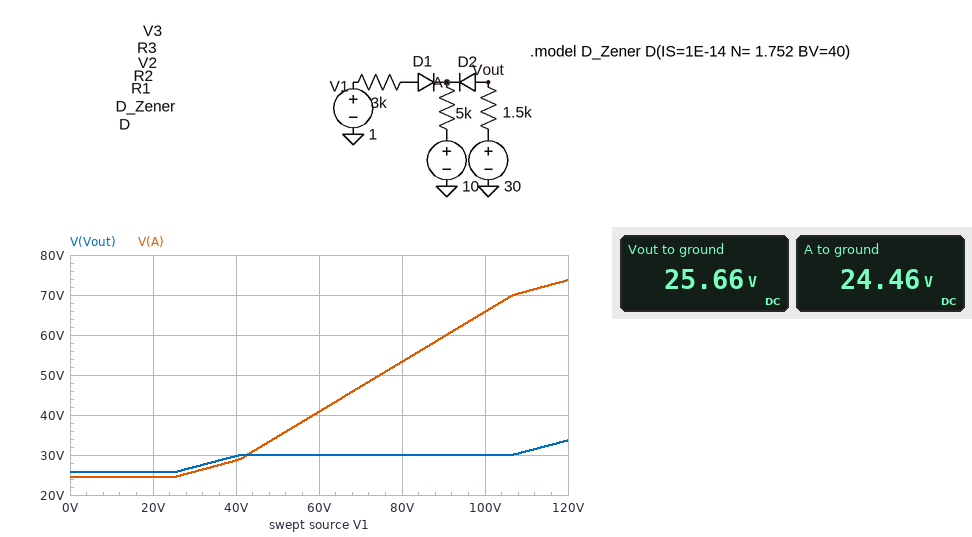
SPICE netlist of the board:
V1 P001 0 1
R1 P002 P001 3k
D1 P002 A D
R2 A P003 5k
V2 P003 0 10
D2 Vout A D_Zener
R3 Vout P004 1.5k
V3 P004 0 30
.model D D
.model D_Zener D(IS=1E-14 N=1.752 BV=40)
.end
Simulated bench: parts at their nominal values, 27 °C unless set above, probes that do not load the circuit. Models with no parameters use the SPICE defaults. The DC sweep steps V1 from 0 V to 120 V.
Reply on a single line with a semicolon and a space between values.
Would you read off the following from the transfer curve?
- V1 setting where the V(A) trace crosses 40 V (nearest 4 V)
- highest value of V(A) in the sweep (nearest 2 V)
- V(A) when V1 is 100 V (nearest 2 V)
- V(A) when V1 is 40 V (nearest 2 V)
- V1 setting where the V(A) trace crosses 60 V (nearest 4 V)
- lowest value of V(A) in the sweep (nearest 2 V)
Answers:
60 V; 74 V; 66 V; 28 V; 92 V; 24 V
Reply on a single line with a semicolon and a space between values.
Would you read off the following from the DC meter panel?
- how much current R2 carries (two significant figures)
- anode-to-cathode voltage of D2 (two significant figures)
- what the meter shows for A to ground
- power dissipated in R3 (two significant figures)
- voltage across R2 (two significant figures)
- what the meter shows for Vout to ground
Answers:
2.9 mA; 1.2 V; 24.46 V; 13 mW; 14 V; 25.66 V
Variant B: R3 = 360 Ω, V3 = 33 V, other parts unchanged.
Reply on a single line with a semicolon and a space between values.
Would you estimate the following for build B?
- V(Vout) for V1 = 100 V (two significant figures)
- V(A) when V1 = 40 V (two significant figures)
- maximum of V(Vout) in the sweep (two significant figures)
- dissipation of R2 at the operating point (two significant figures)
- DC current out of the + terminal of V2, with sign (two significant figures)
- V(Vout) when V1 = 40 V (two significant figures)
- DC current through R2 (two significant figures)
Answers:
33 V; 31 V; 34 V; 83 mW; -4.1 mA; 32 V; 4.1 mA
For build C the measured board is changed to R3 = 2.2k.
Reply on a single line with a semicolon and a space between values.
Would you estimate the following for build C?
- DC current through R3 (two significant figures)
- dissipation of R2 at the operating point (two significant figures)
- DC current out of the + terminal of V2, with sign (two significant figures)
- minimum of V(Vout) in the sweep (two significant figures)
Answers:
2.6 mA; 34 mW; -2.6 mA; 24 V
